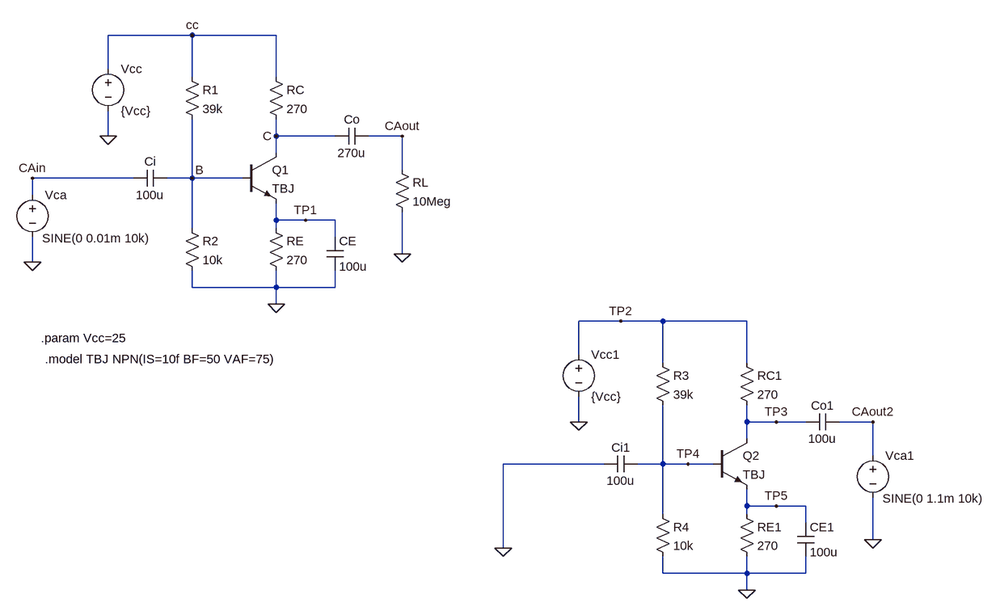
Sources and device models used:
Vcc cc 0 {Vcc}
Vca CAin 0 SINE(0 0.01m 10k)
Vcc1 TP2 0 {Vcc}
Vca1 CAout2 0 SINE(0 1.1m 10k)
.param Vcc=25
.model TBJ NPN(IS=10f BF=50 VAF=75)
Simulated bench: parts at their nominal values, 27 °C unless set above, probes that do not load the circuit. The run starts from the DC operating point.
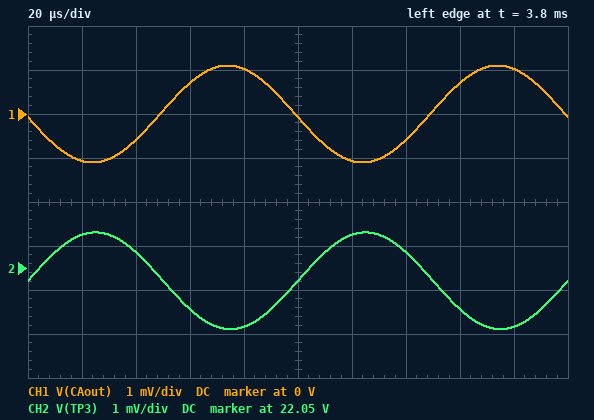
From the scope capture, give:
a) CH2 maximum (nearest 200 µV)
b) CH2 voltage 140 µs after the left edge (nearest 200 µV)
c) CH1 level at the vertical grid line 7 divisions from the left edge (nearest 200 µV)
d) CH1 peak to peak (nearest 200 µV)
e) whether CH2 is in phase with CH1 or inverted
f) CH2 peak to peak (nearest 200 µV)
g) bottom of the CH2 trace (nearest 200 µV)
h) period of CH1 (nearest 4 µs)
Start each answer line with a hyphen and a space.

- 22.0538 V
- 22.0534 V
- -600 µV
- 2.2 mV
- inverted
- 2.2 mV
- 22.0516 V
- 100 µs
